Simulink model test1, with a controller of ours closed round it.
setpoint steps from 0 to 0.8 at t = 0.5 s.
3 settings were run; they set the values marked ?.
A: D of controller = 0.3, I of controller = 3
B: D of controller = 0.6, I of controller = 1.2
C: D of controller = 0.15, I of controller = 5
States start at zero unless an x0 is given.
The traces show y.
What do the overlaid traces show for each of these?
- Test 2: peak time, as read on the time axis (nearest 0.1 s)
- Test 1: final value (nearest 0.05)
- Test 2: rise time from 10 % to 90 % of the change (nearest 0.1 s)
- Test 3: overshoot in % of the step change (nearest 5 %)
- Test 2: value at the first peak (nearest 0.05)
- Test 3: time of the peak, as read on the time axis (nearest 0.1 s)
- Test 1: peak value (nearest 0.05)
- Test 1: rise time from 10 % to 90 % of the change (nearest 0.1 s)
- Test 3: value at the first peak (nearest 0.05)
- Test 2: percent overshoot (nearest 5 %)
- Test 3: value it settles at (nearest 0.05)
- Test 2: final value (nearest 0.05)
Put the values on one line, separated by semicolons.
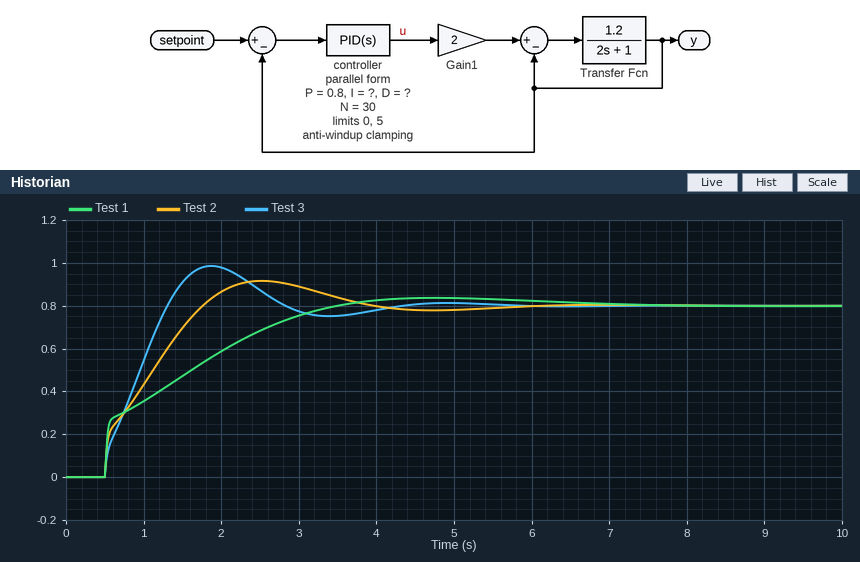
2.5 s; 0.80; 1.0 s; 25 %; 0.90; 1.9 s; 0.85; 2.2 s; 1.00; 15 %; 0.80; 0.80
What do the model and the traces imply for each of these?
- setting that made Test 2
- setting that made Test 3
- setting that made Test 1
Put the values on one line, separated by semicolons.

A; C; B
